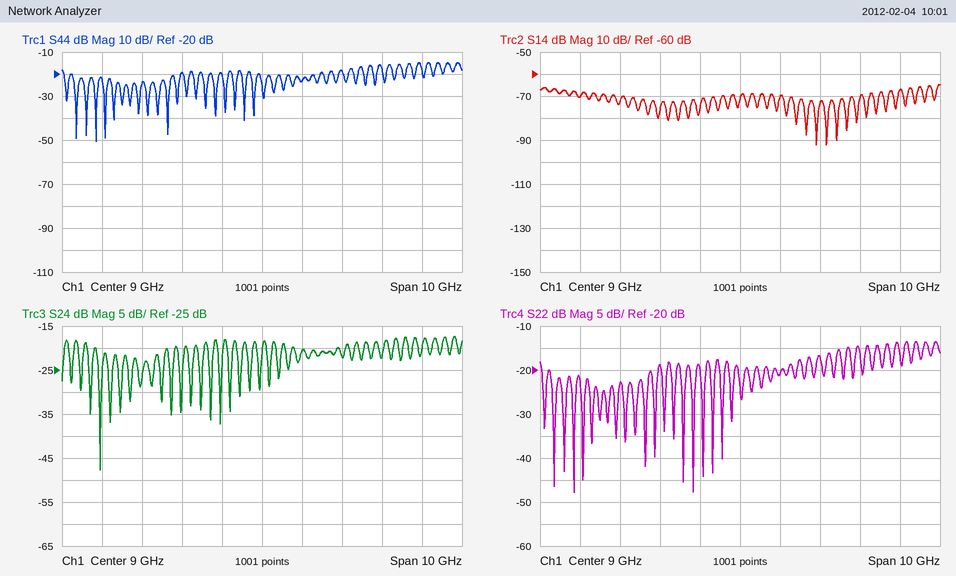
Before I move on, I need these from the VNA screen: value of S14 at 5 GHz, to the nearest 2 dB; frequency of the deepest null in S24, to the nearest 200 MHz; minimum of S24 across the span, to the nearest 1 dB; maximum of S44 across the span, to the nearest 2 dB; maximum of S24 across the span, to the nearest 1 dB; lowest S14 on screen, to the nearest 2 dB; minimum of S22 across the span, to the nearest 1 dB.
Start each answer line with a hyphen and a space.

- -70 dB
- 5.0 GHz
- -48 dB
- -14 dB
- -17 dB
- -92 dB
- -48 dB
